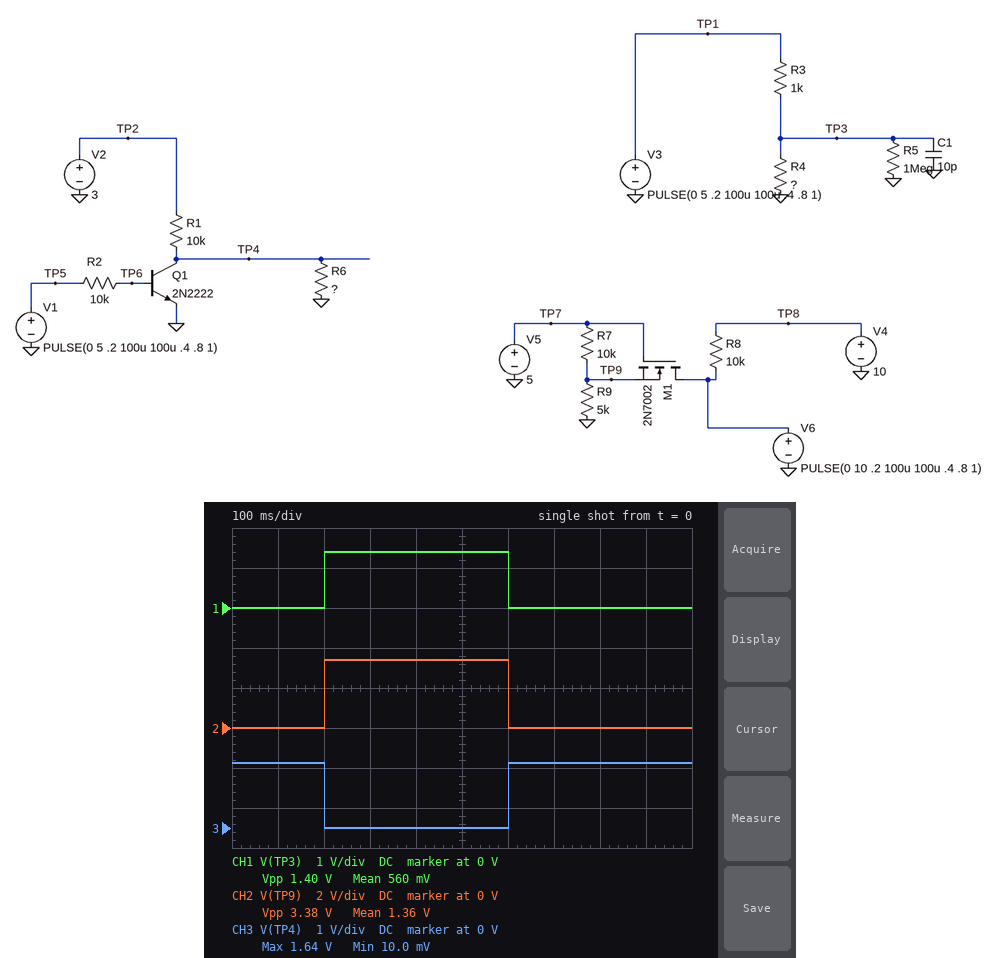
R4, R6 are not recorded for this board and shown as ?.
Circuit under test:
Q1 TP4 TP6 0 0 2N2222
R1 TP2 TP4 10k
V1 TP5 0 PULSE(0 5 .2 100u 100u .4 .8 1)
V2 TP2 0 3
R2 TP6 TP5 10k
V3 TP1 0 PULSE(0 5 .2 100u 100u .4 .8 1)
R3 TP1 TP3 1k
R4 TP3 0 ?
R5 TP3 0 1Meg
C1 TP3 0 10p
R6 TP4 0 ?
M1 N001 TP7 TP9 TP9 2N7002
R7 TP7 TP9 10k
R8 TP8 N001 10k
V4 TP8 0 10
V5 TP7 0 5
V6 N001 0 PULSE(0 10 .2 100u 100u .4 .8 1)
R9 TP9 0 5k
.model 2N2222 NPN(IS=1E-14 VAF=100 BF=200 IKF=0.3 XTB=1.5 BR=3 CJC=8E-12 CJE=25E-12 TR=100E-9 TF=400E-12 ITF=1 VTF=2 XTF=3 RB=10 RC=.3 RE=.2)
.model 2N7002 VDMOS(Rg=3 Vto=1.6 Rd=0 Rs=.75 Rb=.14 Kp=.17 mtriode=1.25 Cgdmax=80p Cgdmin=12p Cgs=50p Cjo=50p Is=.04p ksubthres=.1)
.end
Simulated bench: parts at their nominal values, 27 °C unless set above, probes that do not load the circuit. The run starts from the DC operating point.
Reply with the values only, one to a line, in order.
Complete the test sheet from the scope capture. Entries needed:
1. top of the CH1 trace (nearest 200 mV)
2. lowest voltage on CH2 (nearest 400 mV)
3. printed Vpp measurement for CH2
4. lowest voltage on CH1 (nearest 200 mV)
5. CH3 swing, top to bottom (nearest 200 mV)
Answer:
1.4 V
0 V
3.38 V
0 V
1.6 V
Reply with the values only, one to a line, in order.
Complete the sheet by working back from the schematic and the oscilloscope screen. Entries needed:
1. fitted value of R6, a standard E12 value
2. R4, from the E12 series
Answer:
12 kΩ
390 Ω
